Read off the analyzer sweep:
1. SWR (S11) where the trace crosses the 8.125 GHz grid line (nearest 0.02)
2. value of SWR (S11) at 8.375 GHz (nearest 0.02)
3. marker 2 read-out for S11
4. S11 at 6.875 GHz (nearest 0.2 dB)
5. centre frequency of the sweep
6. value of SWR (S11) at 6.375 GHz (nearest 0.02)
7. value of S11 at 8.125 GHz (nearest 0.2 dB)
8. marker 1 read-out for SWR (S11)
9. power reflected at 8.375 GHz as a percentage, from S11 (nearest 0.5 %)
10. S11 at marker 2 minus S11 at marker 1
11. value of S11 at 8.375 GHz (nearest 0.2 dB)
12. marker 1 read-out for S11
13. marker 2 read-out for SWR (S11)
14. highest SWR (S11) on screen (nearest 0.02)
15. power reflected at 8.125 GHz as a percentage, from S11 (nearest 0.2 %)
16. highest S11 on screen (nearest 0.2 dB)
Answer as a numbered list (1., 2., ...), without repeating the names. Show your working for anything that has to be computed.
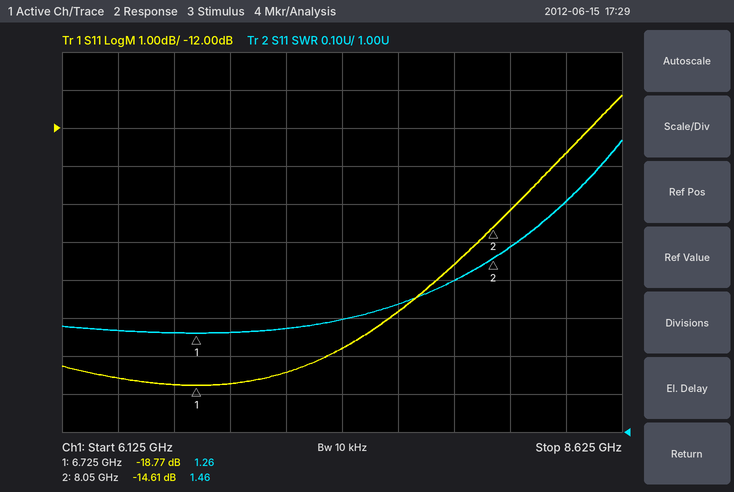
1. 1.48
2. 1.60
3. -14.61 dB
4. -18.8 dB
5. 7.375 GHz
6. 1.26
7. -14.2 dB
8. 1.26
9. 10^(-12.6/10) ≈ 5.5 %
10. -14.61 − (-18.77) = 4.16 dB
11. -12.6 dB
12. -18.77 dB
13. 1.46
14. 1.76
15. 10^(-14.2/10) ≈ 3.8 %
16. -11.2 dB
